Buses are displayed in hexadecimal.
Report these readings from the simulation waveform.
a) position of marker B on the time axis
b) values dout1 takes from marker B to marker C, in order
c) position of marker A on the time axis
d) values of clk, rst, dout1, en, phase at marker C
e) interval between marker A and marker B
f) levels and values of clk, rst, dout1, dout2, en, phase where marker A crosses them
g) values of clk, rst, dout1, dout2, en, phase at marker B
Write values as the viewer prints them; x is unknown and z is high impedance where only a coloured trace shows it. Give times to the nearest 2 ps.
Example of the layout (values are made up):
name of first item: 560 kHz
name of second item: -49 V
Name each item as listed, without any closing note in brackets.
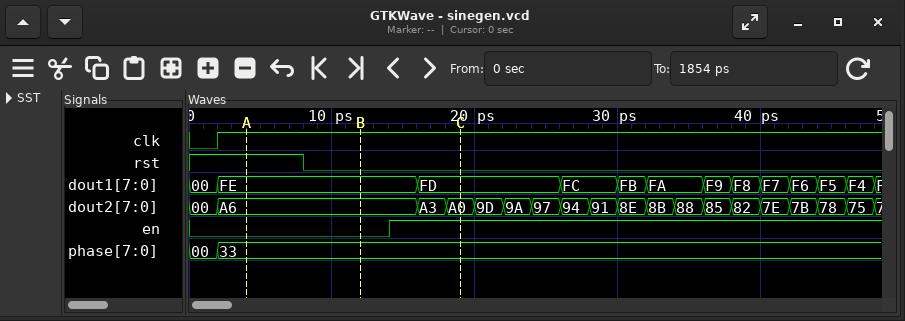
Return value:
position of marker B on the time axis: 12 ps
values dout1 takes from marker B to marker C, in order: FE, FD
position of marker A on the time axis: 4 ps
values of clk, rst, dout1, en, phase at marker C: clk=1, rst=0, dout1=FD, en=1, phase=33
interval between marker A and marker B: 8 ps
levels and values of clk, rst, dout1, dout2, en, phase where marker A crosses them: clk=1, rst=1, dout1=FE, dout2=A6, en=0, phase=33
values of clk, rst, dout1, dout2, en, phase at marker B: clk=1, rst=0, dout1=FE, dout2=A6, en=0, phase=33
